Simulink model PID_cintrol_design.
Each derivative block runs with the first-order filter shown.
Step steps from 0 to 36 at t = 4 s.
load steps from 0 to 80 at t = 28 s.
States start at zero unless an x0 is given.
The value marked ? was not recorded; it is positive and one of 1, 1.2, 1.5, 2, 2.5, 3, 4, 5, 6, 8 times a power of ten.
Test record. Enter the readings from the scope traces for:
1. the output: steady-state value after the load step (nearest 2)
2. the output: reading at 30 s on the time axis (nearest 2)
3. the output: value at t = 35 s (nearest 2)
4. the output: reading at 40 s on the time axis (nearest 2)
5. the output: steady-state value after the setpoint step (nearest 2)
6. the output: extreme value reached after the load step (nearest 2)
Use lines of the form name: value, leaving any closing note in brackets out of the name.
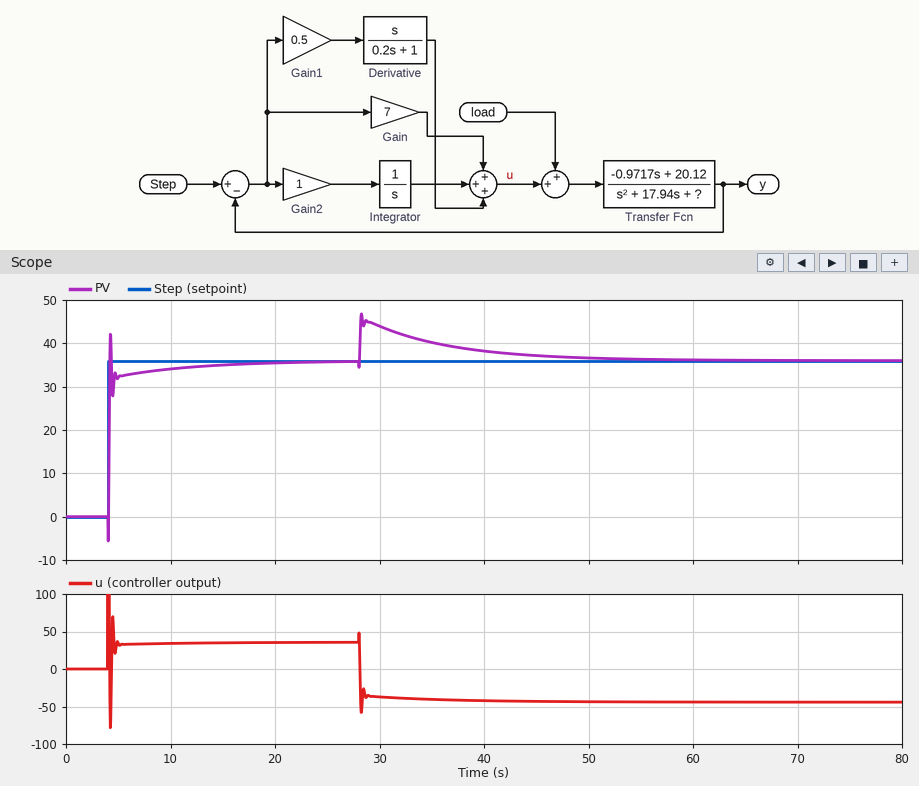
the output: steady-state value after the load step: 36
the output: reading at 30 s on the time axis: 44
the output: value at t = 35 s: 40
the output: reading at 40 s on the time axis: 38
the output: steady-state value after the setpoint step: 36
the output: extreme value reached after the load step: 46
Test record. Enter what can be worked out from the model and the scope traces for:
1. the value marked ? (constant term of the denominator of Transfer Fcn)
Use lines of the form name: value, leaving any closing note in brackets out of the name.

the value marked ?: 20
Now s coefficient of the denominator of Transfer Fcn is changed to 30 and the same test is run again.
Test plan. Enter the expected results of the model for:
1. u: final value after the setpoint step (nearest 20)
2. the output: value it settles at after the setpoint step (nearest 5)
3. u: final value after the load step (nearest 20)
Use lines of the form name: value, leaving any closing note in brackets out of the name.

u: final value after the setpoint step: 40
the output: value it settles at after the setpoint step: 35
u: final value after the load step: -40
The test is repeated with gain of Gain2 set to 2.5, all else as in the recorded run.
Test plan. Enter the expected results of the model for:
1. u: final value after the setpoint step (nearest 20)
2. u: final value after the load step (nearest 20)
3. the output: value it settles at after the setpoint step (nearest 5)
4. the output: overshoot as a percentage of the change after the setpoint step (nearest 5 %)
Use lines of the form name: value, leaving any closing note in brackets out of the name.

u: final value after the setpoint step: 40
u: final value after the load step: -40
the output: value it settles at after the setpoint step: 35
the output: overshoot as a percentage of the change after the setpoint step: 20 %
